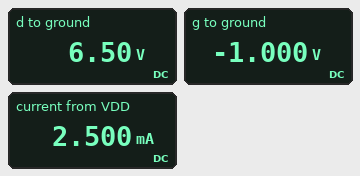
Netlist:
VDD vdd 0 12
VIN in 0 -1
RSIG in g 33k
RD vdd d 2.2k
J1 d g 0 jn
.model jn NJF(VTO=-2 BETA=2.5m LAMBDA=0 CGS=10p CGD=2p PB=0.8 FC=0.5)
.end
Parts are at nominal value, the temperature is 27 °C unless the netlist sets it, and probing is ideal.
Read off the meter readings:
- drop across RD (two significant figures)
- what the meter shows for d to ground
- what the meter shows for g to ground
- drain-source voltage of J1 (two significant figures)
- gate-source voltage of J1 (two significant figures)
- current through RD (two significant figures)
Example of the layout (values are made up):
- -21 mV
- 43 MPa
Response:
- 5.5 V
- 6.50 V
- -1.000 V
- 6.5 V
- -1.0 V
- 2.5 mA
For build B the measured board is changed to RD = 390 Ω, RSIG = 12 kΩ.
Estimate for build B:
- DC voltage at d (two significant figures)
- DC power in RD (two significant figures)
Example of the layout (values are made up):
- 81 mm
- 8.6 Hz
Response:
- 11 V
- 2.4 mW
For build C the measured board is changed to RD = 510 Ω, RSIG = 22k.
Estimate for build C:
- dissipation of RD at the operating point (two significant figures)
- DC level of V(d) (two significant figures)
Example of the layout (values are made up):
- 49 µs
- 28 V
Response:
- 3.2 mW
- 11 V
